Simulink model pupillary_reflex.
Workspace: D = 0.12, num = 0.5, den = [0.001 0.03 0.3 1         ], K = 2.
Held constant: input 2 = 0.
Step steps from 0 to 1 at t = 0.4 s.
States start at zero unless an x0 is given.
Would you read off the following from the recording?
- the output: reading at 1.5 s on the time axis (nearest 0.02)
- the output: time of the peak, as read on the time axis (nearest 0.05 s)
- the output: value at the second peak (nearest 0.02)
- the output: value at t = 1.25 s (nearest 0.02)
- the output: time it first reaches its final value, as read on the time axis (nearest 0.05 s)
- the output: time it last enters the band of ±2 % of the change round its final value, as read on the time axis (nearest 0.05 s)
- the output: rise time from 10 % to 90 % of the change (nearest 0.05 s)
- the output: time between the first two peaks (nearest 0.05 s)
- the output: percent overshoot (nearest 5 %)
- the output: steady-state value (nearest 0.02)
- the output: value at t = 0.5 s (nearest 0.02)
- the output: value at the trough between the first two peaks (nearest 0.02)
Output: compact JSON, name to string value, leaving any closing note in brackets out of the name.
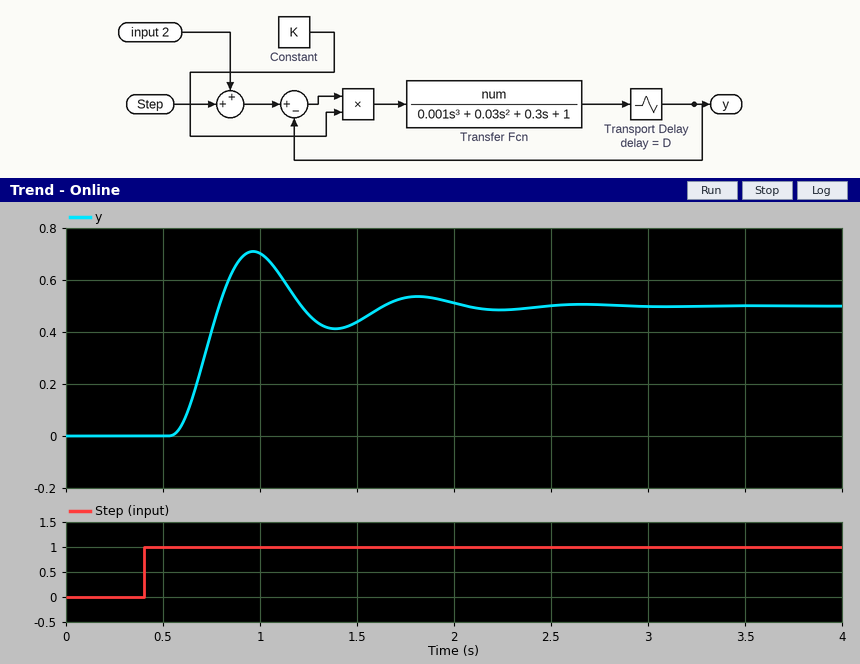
{"the output: reading at 1.5 s on the time axis": "0.44", "the output: time of the peak, as read on the time axis": "0.95 s", "the output: value at the second peak": "0.54", "the output: value at t = 1.25 s": "0.46", "the output: time it first reaches its final value, as read on the time axis": "0.80 s", "the output: time it last enters the band of ±2 % of the change round its final value, as read on the time axis": "2.35 s", "the output: rise time from 10 % to 90 % of the change": "0.15 s", "the output: time between the first two peaks": "0.85 s", "the output: percent overshoot": "40 %", "the output: steady-state value": "0.50", "the output: value at t = 0.5 s": "0.00", "the output: value at the trough between the first two peaks": "0.42"}
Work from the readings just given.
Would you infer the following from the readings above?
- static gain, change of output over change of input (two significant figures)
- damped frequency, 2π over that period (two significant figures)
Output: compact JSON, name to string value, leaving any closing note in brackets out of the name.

{"static gain, change of output over change of input": "0.50", "damped frequency, 2π over that period": "7.4 rad/s"}
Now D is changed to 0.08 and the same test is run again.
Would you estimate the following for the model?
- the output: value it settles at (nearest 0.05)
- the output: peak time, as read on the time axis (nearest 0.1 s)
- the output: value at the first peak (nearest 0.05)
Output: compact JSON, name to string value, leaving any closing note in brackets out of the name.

{"the output: value it settles at": "0.50", "the output: peak time, as read on the time axis": "0.9 s", "the output: value at the first peak": "0.65"}
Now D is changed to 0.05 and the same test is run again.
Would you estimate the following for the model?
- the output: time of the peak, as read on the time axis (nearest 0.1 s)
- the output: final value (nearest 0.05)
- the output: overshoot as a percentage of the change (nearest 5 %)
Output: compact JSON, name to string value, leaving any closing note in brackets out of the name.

{"the output: time of the peak, as read on the time axis": "0.9 s", "the output: final value": "0.50", "the output: overshoot as a percentage of the change": "25 %"}
